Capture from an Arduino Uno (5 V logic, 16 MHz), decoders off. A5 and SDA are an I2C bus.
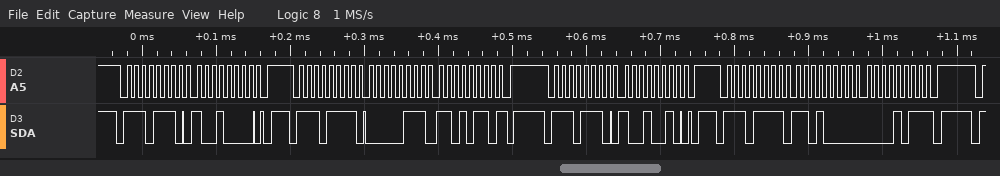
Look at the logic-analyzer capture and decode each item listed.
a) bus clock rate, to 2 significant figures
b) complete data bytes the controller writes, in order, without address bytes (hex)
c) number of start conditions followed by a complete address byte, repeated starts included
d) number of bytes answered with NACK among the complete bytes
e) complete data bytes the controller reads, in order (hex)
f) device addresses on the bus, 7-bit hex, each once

100 kHz
90 92
4
2
07 D6 D0 0B
0x77
